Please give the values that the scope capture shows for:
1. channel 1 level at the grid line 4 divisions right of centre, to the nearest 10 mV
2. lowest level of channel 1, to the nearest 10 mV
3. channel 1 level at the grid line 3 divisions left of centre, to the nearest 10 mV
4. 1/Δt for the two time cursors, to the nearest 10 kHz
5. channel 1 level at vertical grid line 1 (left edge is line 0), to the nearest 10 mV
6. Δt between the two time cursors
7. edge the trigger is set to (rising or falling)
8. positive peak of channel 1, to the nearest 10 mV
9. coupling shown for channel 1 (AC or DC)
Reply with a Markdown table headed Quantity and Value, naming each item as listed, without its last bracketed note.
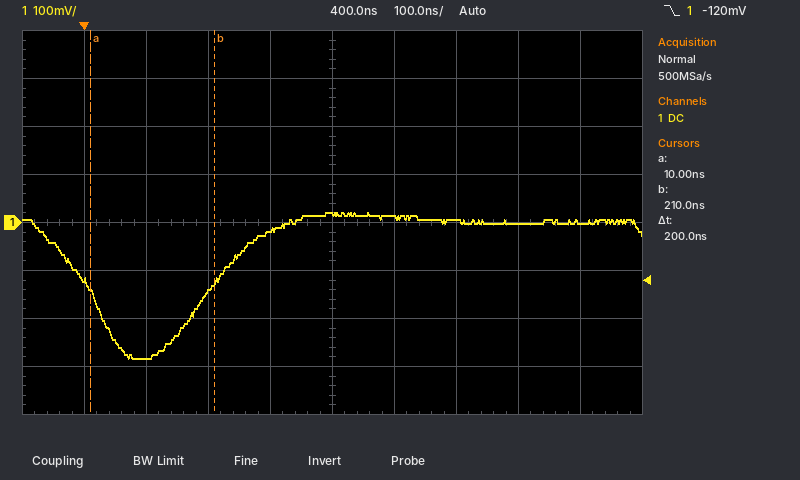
| Quantity | Value |
|---|---|
| channel 1 level at the grid line 4 divisions right of centre, to the nearest 10 mV | 0 mV |
| lowest level of channel 1, to the nearest 10 mV | -280 mV |
| channel 1 level at the grid line 3 divisions left of centre, to the nearest 10 mV | -280 mV |
| 1/Δt for the two time cursors, to the nearest 10 kHz | 5.00 MHz |
| channel 1 level at vertical grid line 1 (left edge is line 0), to the nearest 10 mV | -120 mV |
| Δt between the two time cursors | 200 ns |
| edge the trigger is set to | falling |
| positive peak of channel 1, to the nearest 10 mV | 20 mV |
| coupling shown for channel 1 | DC |
